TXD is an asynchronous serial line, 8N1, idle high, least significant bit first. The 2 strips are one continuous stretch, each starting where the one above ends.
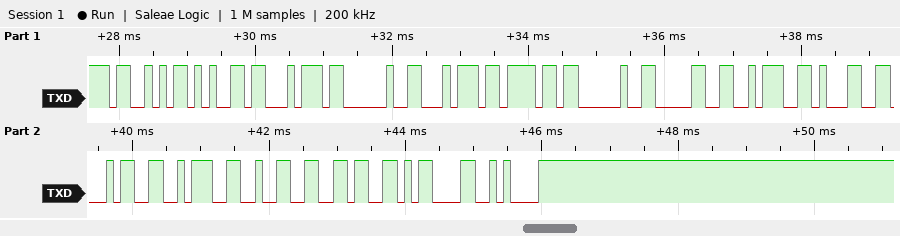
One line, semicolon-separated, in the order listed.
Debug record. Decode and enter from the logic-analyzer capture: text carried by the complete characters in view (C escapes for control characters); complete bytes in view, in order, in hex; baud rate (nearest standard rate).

"Set to 0:14:26\r\n"; 53 65 74 20 74 6F 20 30 3A 31 34 3A 32 36 0D 0A; 9600 baud
